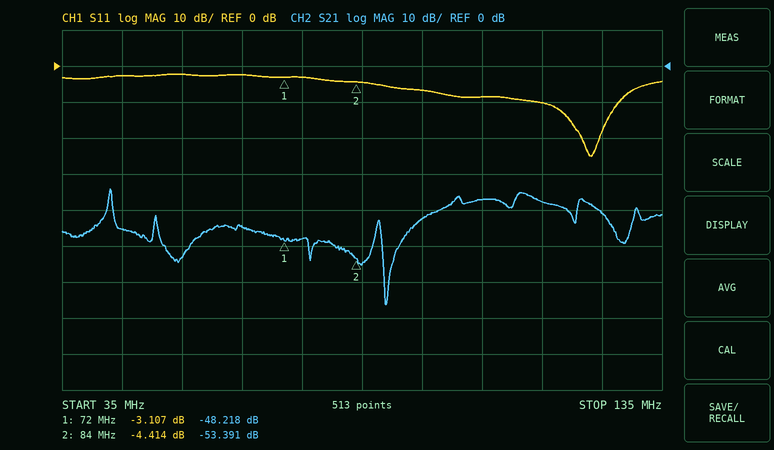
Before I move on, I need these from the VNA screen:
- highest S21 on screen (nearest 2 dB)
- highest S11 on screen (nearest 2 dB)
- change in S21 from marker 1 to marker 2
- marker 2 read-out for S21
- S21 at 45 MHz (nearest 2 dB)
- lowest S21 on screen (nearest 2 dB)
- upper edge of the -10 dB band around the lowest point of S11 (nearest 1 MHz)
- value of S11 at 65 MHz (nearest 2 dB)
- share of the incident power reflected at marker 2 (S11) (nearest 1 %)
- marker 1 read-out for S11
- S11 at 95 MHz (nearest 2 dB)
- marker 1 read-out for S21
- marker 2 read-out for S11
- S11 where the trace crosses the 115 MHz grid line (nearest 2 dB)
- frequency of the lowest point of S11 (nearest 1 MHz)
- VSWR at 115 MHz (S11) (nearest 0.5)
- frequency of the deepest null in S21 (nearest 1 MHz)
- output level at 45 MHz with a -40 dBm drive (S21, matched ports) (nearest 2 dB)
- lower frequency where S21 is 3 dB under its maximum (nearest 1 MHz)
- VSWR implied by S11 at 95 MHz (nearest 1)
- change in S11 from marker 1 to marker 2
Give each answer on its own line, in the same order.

-34 dB
-2 dB
-5.173 dB
-53.391 dB
-46 dB
-66 dB
128 MHz
-2 dB
36 %
-3.107 dB
-6 dB
-48.218 dB
-4.414 dB
-10 dB
123 MHz
2.0
89 MHz
-86 dBm
43 MHz
3
-1.307 dB
